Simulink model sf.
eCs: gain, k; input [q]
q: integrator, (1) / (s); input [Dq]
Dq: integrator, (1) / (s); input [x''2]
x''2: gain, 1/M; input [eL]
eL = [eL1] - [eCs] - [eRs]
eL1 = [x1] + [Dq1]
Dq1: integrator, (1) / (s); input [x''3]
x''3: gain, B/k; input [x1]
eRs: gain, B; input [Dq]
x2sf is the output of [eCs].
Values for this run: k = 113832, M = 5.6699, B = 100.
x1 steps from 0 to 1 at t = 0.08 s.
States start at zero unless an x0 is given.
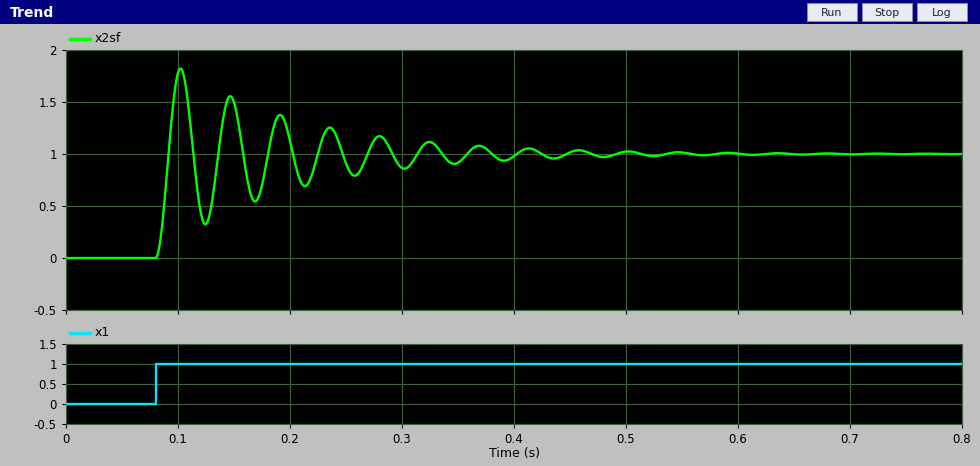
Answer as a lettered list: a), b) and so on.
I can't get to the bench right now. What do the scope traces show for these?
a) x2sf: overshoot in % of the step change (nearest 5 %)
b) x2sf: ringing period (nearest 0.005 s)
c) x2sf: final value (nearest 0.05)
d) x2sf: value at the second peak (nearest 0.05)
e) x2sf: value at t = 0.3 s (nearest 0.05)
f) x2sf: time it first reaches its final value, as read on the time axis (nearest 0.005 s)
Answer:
a) 80 %
b) 0.045 s
c) 1.00
d) 1.55
e) 0.85
f) 0.090 s
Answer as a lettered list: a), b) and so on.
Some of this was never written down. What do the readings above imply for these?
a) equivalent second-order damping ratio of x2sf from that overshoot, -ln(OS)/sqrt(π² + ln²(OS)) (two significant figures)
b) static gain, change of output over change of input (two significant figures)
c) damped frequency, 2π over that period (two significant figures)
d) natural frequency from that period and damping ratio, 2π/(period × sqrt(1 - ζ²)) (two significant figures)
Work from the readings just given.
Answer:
a) 0.071
b) 1.0
c) 140 rad/s
d) 140 rad/s
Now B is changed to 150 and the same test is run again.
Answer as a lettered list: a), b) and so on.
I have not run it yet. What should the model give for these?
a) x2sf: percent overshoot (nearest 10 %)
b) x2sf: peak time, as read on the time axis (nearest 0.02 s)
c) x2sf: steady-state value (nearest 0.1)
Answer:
a) 70 %
b) 0.10 s
c) 1.0
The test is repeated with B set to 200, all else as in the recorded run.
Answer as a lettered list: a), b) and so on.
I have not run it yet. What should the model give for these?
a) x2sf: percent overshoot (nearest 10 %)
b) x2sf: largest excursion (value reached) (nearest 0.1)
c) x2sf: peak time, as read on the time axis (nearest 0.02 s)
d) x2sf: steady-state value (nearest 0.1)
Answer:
a) 70 %
b) 1.7
c) 0.10 s
d) 1.0
